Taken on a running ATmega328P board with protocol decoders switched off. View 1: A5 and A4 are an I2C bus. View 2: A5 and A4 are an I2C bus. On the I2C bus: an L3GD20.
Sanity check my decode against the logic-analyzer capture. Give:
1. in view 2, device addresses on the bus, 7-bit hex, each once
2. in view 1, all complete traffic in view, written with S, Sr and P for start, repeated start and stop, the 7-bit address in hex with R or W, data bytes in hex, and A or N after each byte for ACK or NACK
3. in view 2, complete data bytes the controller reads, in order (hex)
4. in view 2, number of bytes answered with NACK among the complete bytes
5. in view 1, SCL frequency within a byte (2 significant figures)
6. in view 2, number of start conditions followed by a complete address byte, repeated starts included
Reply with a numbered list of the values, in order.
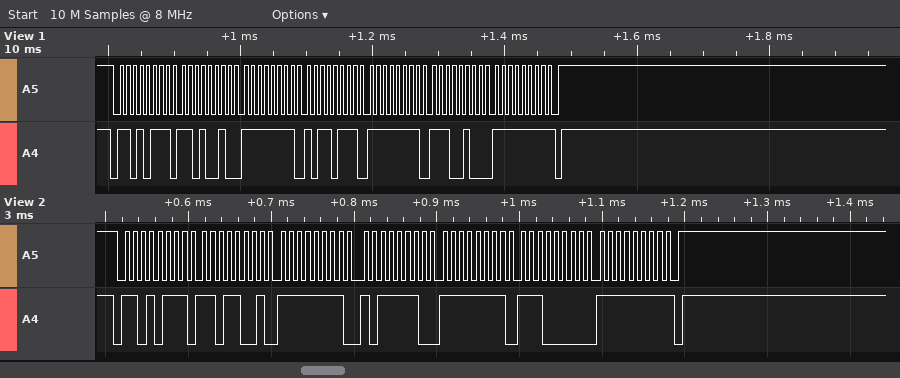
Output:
1. 0x6B
2. S 6BR A D2 A FF A B7 A FF A E4 A FF N P
3. D9 FF BE FF E0 FF
4. 1
5. 100 kHz
6. 1
